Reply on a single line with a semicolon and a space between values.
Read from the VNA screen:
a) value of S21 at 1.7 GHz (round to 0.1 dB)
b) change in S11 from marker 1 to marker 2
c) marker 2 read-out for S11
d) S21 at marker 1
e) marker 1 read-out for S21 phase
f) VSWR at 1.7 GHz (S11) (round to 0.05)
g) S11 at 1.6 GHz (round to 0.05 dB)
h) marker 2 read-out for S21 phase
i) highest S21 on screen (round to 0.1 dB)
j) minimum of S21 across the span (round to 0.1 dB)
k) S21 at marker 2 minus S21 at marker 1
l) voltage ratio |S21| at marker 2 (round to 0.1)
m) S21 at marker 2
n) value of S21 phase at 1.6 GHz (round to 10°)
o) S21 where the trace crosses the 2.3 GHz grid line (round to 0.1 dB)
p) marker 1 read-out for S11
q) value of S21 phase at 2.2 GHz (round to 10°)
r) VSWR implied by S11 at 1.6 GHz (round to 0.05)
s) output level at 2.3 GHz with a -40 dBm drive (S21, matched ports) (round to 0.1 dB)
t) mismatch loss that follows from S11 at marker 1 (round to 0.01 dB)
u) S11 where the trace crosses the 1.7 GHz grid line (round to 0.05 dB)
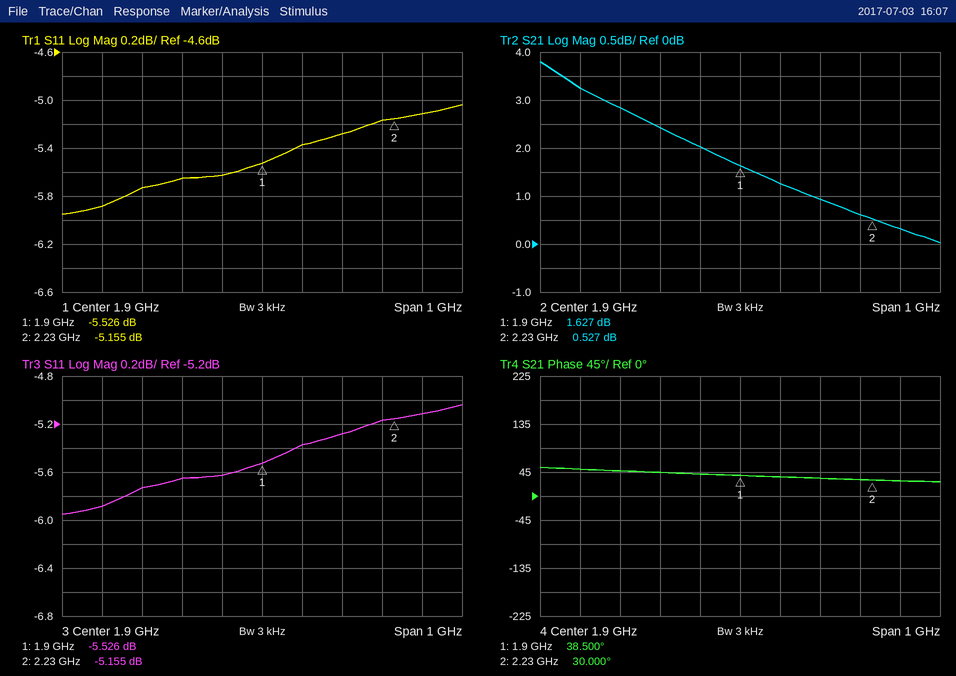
2.4 dB; 0.371 dB; -5.155 dB; 1.627 dB; 38.500°; 3.20; -5.75 dB; 30.000°; 3.8 dB; 0.0 dB; -1.100 dB; 1.1; 0.527 dB; 50°; 0.3 dB; -5.526 dB; 30°; 3.15; -39.7 dBm; 1.43 dB; -5.65 dB
